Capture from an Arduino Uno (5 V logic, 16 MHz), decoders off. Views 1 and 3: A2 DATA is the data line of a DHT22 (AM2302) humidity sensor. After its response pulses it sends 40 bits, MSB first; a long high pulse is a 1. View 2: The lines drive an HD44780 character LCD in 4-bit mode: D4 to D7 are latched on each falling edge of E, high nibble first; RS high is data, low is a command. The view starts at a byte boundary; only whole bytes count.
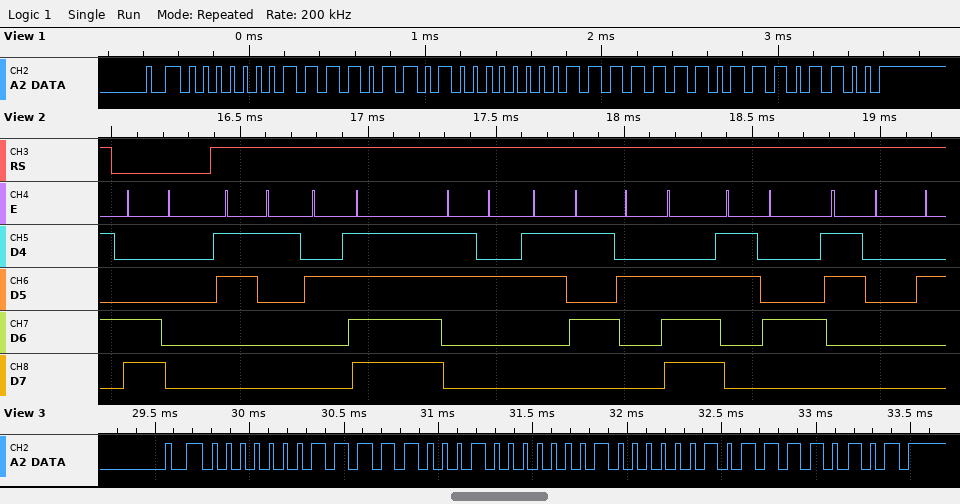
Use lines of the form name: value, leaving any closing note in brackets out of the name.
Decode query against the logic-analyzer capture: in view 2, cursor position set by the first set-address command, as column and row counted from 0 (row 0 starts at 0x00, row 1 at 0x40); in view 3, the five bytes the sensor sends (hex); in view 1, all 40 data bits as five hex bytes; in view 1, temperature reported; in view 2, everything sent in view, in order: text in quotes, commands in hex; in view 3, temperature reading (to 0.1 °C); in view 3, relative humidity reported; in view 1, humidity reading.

in view 2, cursor position set by the first set-address command, as column and row counted from 0: column 0, row 1
in view 3, the five bytes the sensor sends: 01 F1 01 02 F5
in view 1, all 40 data bits as five hex bytes: 01 ED 00 FE EC
in view 1, temperature reported: 25.4 °C
in view 2, everything sent in view, in order: text in quotes, commands in hex: 0xC0 "1/25.40"
in view 3, temperature reading: 25.8 °C
in view 3, relative humidity reported: 49.7 %
in view 1, humidity reading: 49.3 %
